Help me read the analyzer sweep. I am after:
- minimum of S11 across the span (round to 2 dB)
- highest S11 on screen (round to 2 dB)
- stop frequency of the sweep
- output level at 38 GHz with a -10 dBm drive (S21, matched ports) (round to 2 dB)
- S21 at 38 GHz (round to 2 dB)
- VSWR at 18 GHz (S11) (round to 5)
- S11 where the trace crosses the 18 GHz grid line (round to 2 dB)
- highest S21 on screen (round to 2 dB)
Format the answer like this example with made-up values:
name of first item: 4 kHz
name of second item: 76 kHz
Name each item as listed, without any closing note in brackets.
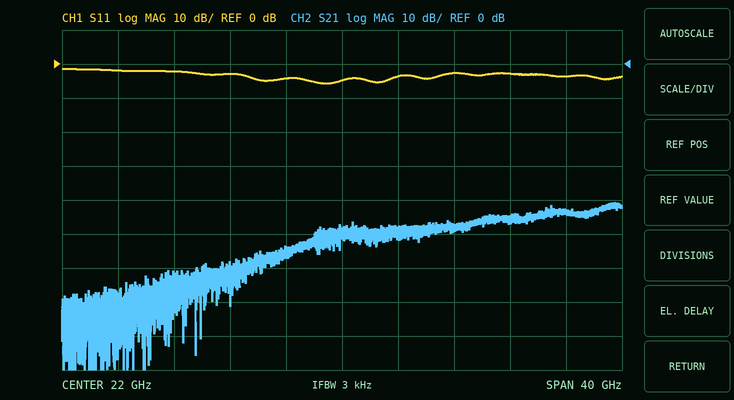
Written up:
minimum of S11 across the span: -6 dB
highest S11 on screen: -2 dB
stop frequency of the sweep: 42 GHz
output level at 38 GHz with a -10 dBm drive (S21, matched ports): -54 dBm
S21 at 38 GHz: -44 dB
VSWR at 18 GHz (S11): 5
S11 where the trace crosses the 18 GHz grid line: -4 dB
highest S21 on screen: -40 dB
